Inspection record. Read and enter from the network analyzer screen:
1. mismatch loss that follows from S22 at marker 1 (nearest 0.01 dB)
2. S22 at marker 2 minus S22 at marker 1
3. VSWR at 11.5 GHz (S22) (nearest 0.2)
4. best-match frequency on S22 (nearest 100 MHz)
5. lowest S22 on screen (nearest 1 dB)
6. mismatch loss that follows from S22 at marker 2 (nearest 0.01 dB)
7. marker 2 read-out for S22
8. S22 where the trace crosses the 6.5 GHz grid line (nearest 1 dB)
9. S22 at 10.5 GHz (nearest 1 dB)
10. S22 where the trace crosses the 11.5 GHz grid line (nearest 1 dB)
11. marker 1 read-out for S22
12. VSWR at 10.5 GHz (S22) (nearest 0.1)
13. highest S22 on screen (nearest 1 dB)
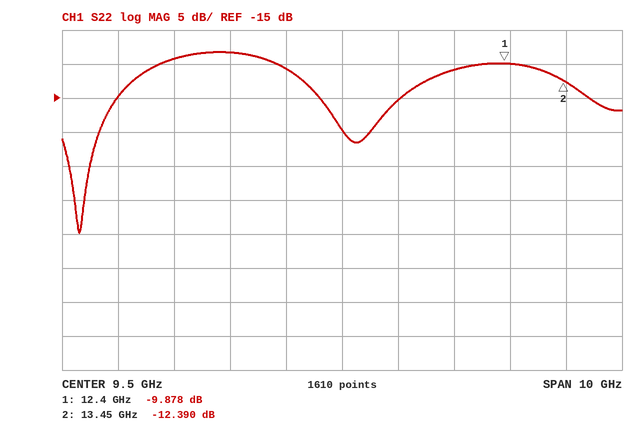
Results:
0.47 dB
-2.512 dB
1.8
4.8 GHz
-35 dB
0.26 dB
-12.390 dB
-9 dB
-15 dB
-11 dB
-9.878 dB
1.4
-8 dB
